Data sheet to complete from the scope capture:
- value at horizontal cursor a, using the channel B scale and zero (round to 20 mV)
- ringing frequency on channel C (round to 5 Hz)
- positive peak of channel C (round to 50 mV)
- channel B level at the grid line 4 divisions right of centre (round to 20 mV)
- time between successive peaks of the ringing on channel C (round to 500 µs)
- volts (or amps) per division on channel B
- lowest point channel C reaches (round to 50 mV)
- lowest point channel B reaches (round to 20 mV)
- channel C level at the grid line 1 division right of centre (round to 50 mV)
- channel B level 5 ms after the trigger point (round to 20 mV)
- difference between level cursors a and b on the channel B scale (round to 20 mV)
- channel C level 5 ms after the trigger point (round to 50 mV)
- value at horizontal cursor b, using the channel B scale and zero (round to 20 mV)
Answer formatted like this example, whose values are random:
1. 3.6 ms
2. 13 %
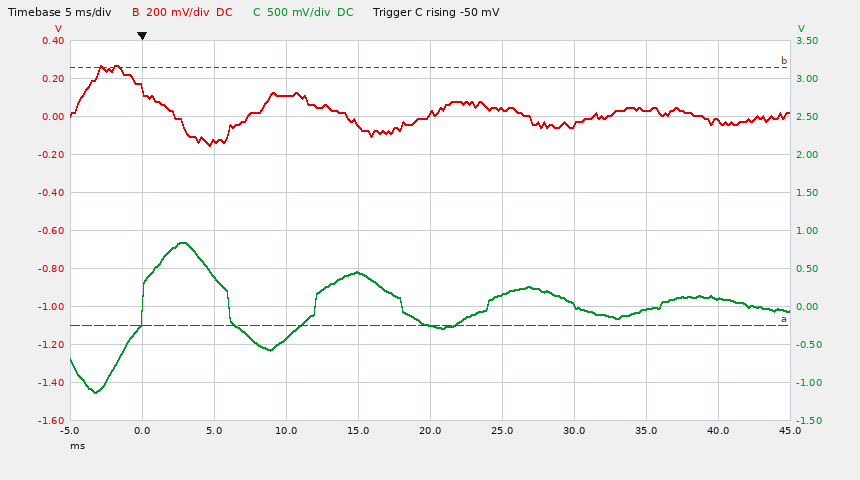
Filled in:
1. -1.10 V
2. 85 Hz
3. 850 mV
4. -20 mV
5. 12.0 ms
6. 200 mV
7. -1.15 V
8. -160 mV
9. 150 mV
10. -140 mV
11. 1.36 V
12. 400 mV
13. 260 mV
